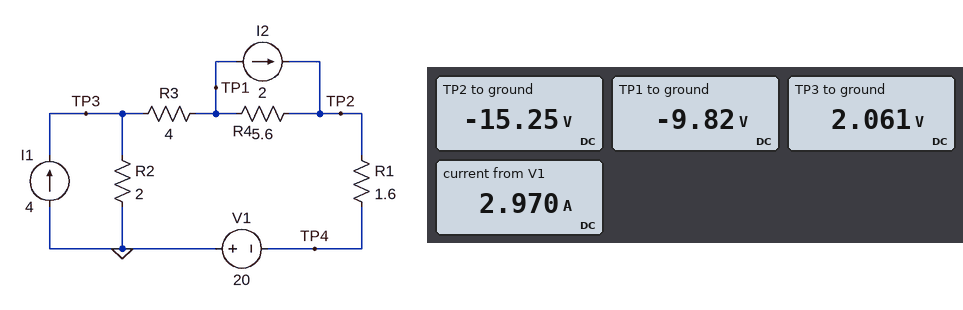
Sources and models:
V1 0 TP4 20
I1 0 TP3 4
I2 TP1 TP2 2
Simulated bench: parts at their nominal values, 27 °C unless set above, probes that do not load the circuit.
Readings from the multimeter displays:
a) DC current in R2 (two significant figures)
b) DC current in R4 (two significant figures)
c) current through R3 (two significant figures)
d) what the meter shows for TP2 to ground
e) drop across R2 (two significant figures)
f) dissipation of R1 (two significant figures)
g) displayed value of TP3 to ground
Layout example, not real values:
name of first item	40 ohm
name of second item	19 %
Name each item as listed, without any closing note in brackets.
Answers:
DC current in R2	1.0 A
DC current in R4	970 mA
current through R3	3.0 A
what the meter shows for TP2 to ground	-15.25 V
drop across R2	2.1 V
dissipation of R1	14 W
displayed value of TP3 to ground	2.061 V
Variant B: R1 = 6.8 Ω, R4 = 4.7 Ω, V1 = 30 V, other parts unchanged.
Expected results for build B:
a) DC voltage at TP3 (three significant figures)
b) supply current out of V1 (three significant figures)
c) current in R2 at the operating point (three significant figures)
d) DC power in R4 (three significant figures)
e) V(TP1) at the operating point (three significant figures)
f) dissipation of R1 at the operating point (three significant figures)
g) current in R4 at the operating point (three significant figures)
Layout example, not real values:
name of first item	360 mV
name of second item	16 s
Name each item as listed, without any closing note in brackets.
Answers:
DC voltage at TP3	2.58 V
supply current out of V1	2.71 A
current in R2 at the operating point	1.29 A
DC power in R4	2.36 W
V(TP1) at the operating point	-8.25 V
dissipation of R1 at the operating point	49.9 W
current in R4 at the operating point	709 mA
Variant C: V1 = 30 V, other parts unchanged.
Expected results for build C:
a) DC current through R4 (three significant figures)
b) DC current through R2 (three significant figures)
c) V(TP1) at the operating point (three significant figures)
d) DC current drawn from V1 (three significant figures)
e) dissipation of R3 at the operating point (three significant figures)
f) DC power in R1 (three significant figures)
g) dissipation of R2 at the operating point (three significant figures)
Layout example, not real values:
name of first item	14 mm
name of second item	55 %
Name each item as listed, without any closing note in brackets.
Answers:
DC current through R4	1.73 A
DC current through R2	273 mA
V(TP1) at the operating point	-14.4 V
DC current drawn from V1	3.73 A
dissipation of R3 at the operating point	55.6 W
DC power in R1	22.2 W
dissipation of R2 at the operating point	149 mW
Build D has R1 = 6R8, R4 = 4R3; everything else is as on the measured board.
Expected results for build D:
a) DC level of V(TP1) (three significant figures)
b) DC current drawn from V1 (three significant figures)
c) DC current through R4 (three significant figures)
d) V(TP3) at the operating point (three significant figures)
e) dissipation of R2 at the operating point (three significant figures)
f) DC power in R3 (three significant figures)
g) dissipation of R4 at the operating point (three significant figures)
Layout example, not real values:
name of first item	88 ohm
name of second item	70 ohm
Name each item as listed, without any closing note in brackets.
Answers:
DC level of V(TP1)	-4.84 V
DC current drawn from V1	2.14 A
DC current through R4	140 mA
V(TP3) at the operating point	3.72 V
dissipation of R2 at the operating point	6.92 W
DC power in R3	18.3 W
dissipation of R4 at the operating point	84.7 mW
